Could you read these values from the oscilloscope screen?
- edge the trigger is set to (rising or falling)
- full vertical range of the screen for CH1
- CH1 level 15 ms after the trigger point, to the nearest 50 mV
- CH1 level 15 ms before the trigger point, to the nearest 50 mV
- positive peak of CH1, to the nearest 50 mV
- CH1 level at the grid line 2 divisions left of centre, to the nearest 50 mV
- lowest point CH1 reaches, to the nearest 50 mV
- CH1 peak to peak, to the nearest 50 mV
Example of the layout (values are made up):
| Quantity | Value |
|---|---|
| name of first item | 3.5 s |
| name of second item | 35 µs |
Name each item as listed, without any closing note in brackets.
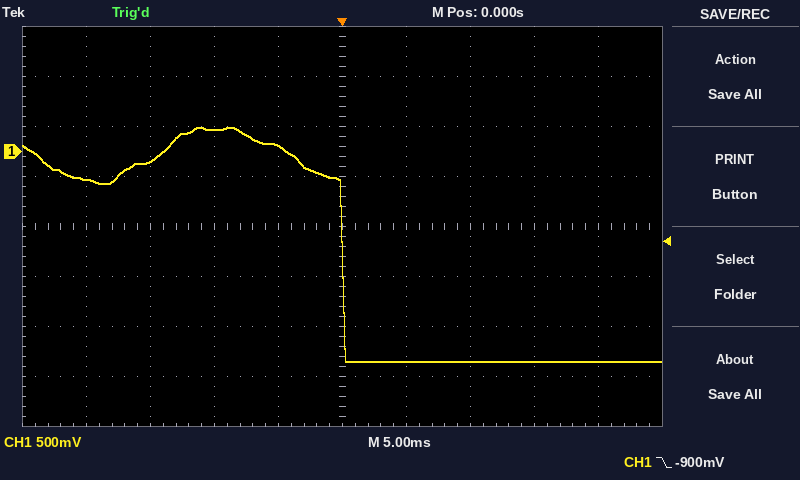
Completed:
| Quantity | Value |
|---|---|
| edge the trigger is set to | falling |
| full vertical range of the screen for CH1 | 4 V |
| CH1 level 15 ms after the trigger point, to the nearest 50 mV | -2.10 V |
| CH1 level 15 ms before the trigger point, to the nearest 50 mV | -100 mV |
| positive peak of CH1, to the nearest 50 mV | 250 mV |
| CH1 level at the grid line 2 divisions left of centre, to the nearest 50 mV | 200 mV |
| lowest point CH1 reaches, to the nearest 50 mV | -2.10 V |
| CH1 peak to peak, to the nearest 50 mV | 2.35 V |
